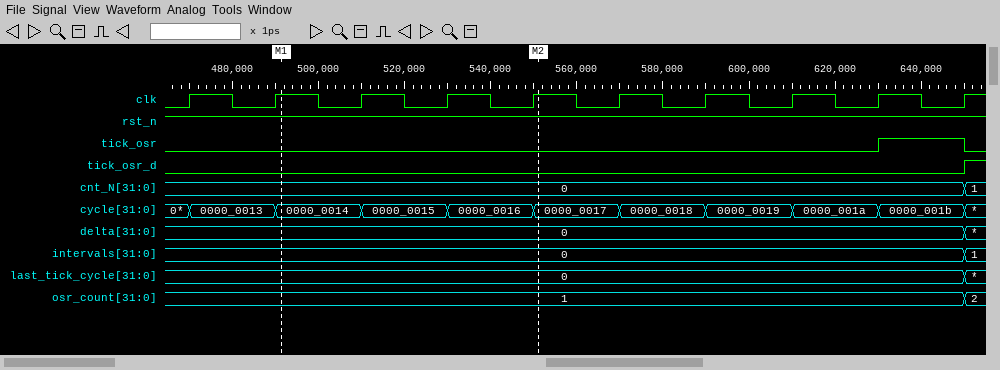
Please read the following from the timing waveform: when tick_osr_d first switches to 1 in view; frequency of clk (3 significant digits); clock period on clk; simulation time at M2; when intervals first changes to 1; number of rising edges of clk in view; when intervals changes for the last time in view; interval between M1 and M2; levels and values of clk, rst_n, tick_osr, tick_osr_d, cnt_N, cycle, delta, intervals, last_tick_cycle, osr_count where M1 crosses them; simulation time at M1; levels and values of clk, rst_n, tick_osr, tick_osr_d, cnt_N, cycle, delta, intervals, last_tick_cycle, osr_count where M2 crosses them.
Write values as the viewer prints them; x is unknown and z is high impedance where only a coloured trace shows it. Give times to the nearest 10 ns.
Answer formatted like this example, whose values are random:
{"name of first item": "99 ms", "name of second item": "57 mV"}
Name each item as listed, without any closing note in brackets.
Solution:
{"when tick_osr_d first switches to 1 in view": "650 ns", "frequency of clk": "50.0 MHz", "clock period on clk": "20 ns", "simulation time at M2": "550 ns", "when intervals first changes to 1": "650 ns", "number of rising edges of clk in view": "10", "when intervals changes for the last time in view": "650 ns", "interval between M1 and M2": "60 ns", "levels and values of clk, rst_n, tick_osr, tick_osr_d, cnt_N, cycle, delta, intervals, last_tick_cycle, osr_count where M1 crosses them": "clk=1, rst_n=1, tick_osr=0, tick_osr_d=0, cnt_N=0, cycle=0000_0014, delta=0, intervals=0, last_tick_cycle=0, osr_count=1", "simulation time at M1": "490 ns", "levels and values of clk, rst_n, tick_osr, tick_osr_d, cnt_N, cycle, delta, intervals, last_tick_cycle, osr_count where M2 crosses them": "clk=1, rst_n=1, tick_osr=0, tick_osr_d=0, cnt_N=0, cycle=0000_0017, delta=0, intervals=0, last_tick_cycle=0, osr_count=1"}
